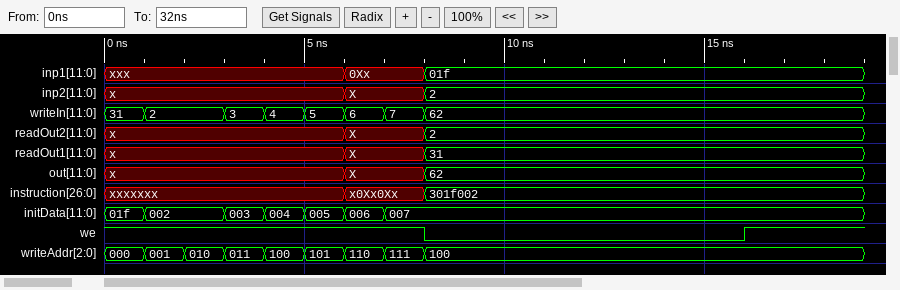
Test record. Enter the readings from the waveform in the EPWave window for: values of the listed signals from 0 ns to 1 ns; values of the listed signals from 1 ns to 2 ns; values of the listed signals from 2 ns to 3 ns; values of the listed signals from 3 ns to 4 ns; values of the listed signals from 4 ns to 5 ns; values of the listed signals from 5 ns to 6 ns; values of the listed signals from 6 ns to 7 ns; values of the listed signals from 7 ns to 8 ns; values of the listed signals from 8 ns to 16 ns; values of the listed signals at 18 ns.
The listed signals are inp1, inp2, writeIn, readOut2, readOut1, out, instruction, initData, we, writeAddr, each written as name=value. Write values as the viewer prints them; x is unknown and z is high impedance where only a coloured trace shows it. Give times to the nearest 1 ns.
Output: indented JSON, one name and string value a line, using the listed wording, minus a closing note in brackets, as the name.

{
  "values of the listed signals from 0 ns to 1 ns": "inp1=xxx, inp2=x, writeIn=31, readOut2=x, readOut1=x, out=x, instruction=xxxxxxx, initData=01f, we=1, writeAddr=000",
  "values of the listed signals from 1 ns to 2 ns": "inp1=xxx, inp2=x, writeIn=2, readOut2=x, readOut1=x, out=x, instruction=xxxxxxx, initData=002, we=1, writeAddr=001",
  "values of the listed signals from 2 ns to 3 ns": "inp1=xxx, inp2=x, writeIn=2, readOut2=x, readOut1=x, out=x, instruction=xxxxxxx, initData=002, we=1, writeAddr=010",
  "values of the listed signals from 3 ns to 4 ns": "inp1=xxx, inp2=x, writeIn=3, readOut2=x, readOut1=x, out=x, instruction=xxxxxxx, initData=003, we=1, writeAddr=011",
  "values of the listed signals from 4 ns to 5 ns": "inp1=xxx, inp2=x, writeIn=4, readOut2=x, readOut1=x, out=x, instruction=xxxxxxx, initData=004, we=1, writeAddr=100",
  "values of the listed signals from 5 ns to 6 ns": "inp1=xxx, inp2=x, writeIn=5, readOut2=x, readOut1=x, out=x, instruction=xxxxxxx, initData=005, we=1, writeAddr=101",
  "values of the listed signals from 6 ns to 7 ns": "inp1=0Xx, inp2=X, writeIn=6, readOut2=X, readOut1=X, out=X, instruction=x0Xx0Xx, initData=006, we=1, writeAddr=110",
  "values of the listed signals from 7 ns to 8 ns": "inp1=0Xx, inp2=X, writeIn=7, readOut2=X, readOut1=X, out=X, instruction=x0Xx0Xx, initData=007, we=1, writeAddr=111",
  "values of the listed signals from 8 ns to 16 ns": "inp1=01f, inp2=2, writeIn=62, readOut2=2, readOut1=31, out=62, instruction=301f002, initData=007, we=0, writeAddr=100",
  "values of the listed signals at 18 ns": "inp1=01f, inp2=2, writeIn=62, readOut2=2, readOut1=31, out=62, instruction=301f002, initData=007, we=1, writeAddr=100"
}
